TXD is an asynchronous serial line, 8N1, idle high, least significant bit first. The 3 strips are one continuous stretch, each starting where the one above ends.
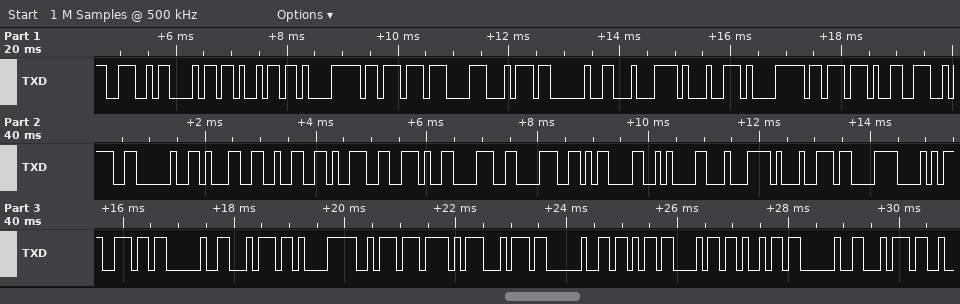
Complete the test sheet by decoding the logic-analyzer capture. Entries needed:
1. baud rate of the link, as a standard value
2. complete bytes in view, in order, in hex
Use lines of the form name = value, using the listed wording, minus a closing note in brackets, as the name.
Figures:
baud rate of the link, as a standard value = 9600 baud
complete bytes in view, in order, in hex = 4E 68 69 E1 BB 87 74 20 C4 91 E1 BB 99 3A 20 31 32 39 2E 38 38 0D 0A C4 91 C3 A8 6E 20 74 E1 BA AF 74 20 6B 68 69 20 74
